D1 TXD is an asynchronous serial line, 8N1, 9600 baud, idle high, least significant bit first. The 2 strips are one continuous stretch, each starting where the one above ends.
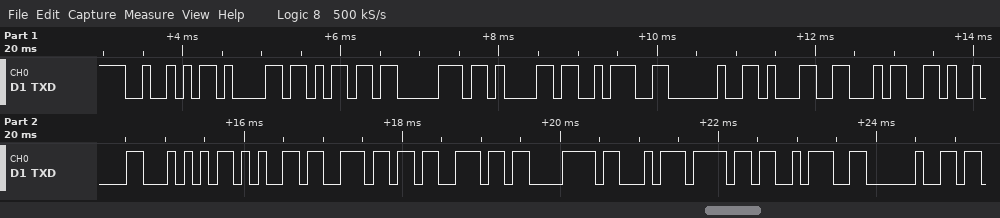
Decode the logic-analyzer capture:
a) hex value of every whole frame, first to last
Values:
0x52 0x61 0x6D 0x70 0x61 0x3A 0x20 0x31 0x34 0x09 0x54 0x65 0x6E 0x73 0xC3 0xA3 0x6F 0x3A 0x20
